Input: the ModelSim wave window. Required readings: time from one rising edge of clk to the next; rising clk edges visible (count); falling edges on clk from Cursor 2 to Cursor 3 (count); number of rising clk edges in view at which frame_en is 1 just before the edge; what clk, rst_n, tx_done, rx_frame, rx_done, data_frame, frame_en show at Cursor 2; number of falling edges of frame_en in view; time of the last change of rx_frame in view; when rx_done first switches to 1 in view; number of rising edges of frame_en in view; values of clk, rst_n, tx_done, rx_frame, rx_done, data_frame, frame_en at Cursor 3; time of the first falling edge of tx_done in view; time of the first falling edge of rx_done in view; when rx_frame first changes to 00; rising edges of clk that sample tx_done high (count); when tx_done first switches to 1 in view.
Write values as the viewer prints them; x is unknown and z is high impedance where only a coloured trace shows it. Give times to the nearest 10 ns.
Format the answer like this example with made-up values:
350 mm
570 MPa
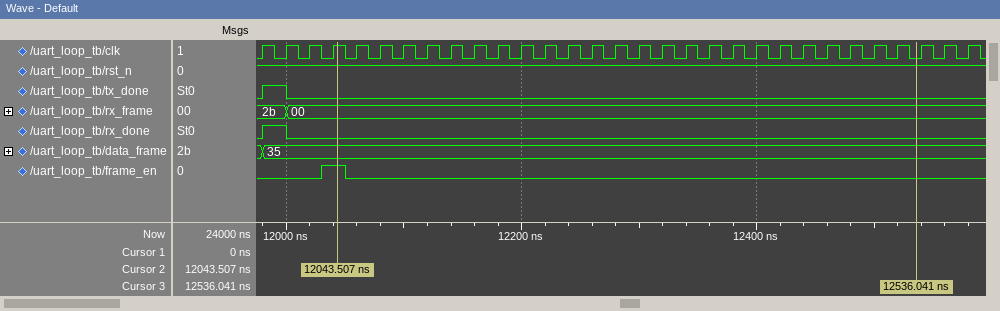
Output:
20 ns
31
25
1
clk=1, rst_n=1, tx_done=0, rx_frame=00, rx_done=0, data_frame=35, frame_en=1
1
12000 ns
11980 ns
1
clk=0, rst_n=1, tx_done=0, rx_frame=00, rx_done=0, data_frame=35, frame_en=0
12000 ns
12000 ns
12000 ns
1
11980 ns
